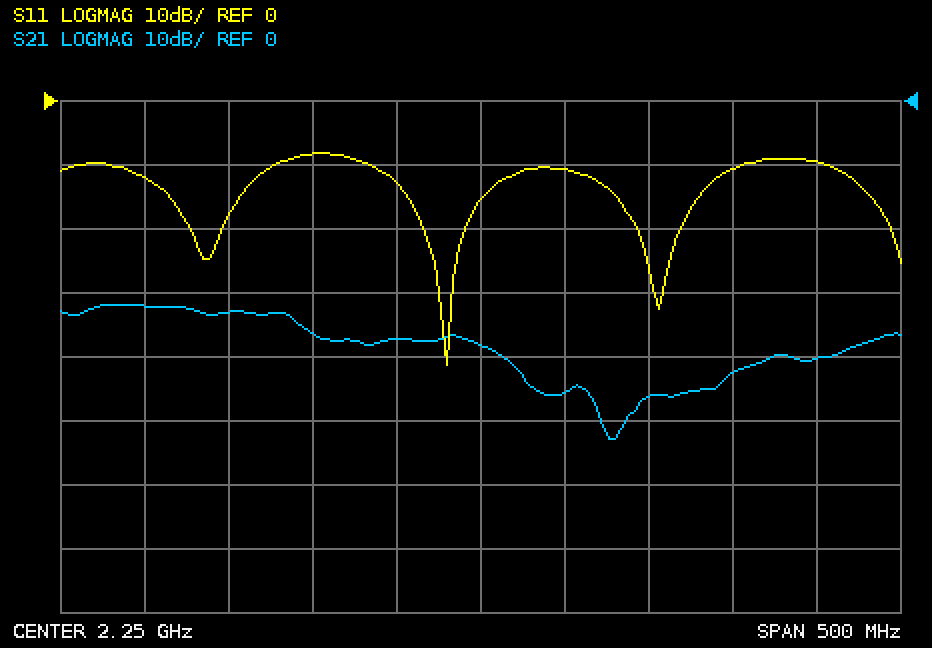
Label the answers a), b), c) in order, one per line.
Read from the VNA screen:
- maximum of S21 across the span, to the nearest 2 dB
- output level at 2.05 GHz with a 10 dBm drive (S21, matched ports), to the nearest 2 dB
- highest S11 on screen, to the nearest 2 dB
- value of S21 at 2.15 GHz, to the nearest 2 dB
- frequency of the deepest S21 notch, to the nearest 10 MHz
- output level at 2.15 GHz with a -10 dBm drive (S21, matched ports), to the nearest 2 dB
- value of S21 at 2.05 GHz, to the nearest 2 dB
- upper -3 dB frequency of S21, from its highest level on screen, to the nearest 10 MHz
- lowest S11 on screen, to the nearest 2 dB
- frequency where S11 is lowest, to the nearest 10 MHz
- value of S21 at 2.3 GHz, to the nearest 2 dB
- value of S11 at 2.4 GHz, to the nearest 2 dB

a) -32 dB
b) -22 dBm
c) -8 dB
d) -36 dB
e) 2.33 GHz
f) -46 dBm
g) -32 dB
h) 2.14 GHz
i) -42 dB
j) 2.23 GHz
k) -46 dB
l) -10 dB
